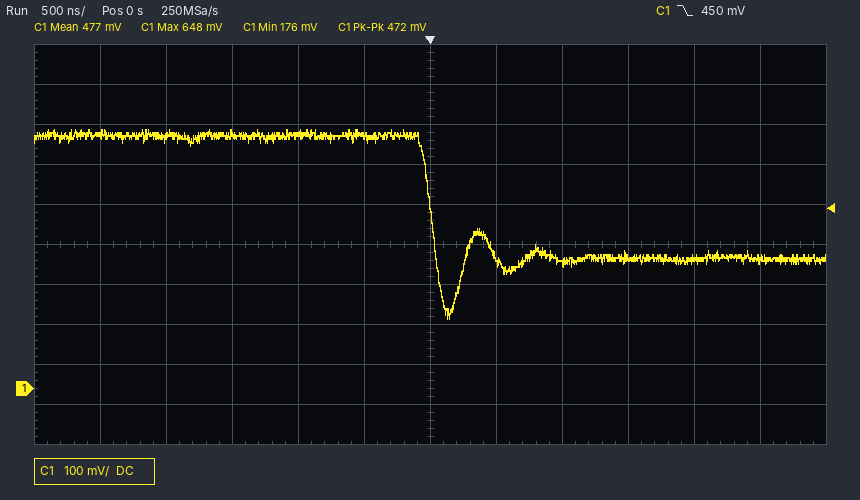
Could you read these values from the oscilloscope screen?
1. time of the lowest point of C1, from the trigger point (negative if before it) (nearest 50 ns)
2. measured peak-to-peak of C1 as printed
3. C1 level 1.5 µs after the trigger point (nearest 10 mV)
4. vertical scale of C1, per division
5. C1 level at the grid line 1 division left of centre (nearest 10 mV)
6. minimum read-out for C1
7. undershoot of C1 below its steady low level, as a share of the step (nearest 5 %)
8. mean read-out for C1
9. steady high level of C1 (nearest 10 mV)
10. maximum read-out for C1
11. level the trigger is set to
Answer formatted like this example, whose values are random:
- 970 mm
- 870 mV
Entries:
- +150 ns
- 472 mV
- 330 mV
- 100 mV
- 630 mV
- 176 mV
- 50 %
- 477 mV
- 630 mV
- 648 mV
- 450 mV
